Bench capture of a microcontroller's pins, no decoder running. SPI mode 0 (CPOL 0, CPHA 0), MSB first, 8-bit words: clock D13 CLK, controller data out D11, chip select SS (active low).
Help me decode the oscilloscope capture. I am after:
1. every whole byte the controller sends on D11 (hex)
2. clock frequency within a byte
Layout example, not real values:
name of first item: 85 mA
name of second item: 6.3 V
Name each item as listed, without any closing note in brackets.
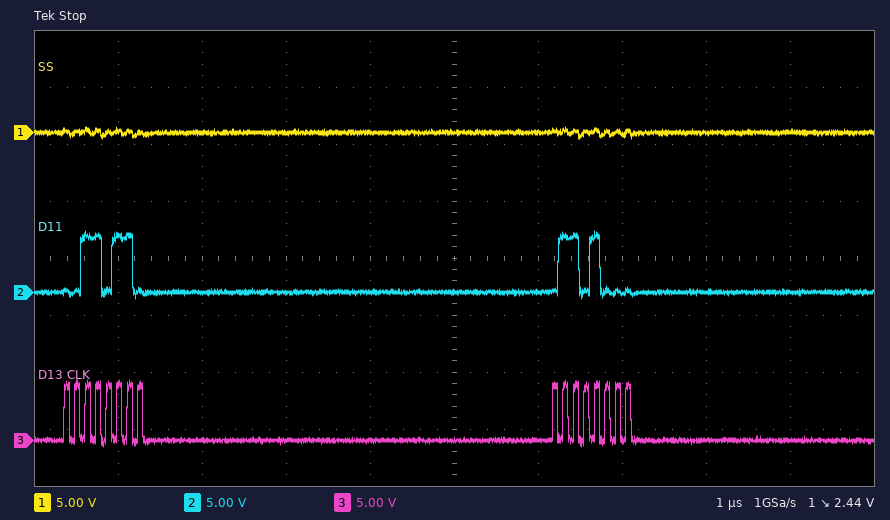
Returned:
every whole byte the controller sends on D11: 36 68
clock frequency within a byte: 8 MHz
